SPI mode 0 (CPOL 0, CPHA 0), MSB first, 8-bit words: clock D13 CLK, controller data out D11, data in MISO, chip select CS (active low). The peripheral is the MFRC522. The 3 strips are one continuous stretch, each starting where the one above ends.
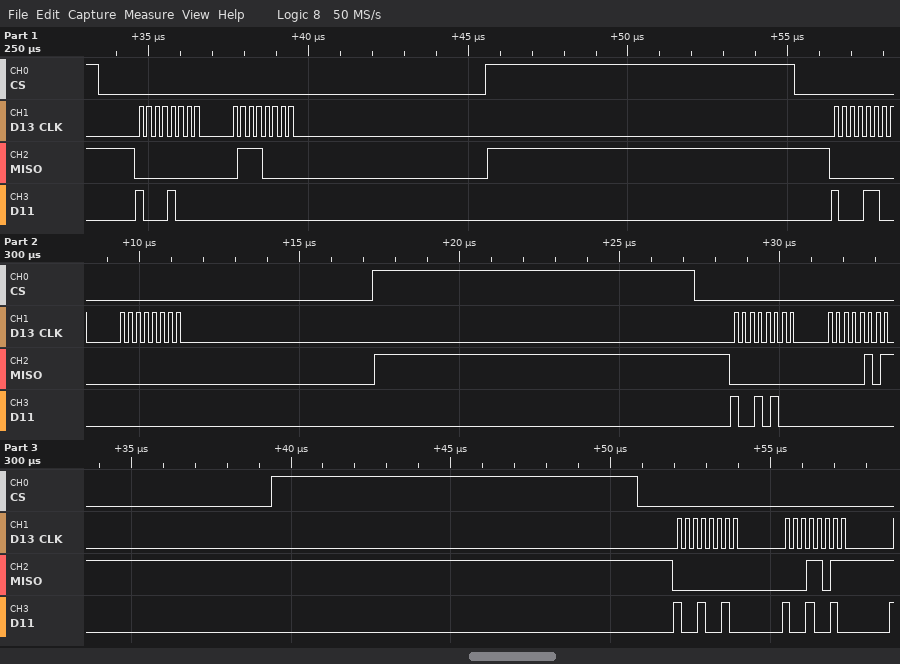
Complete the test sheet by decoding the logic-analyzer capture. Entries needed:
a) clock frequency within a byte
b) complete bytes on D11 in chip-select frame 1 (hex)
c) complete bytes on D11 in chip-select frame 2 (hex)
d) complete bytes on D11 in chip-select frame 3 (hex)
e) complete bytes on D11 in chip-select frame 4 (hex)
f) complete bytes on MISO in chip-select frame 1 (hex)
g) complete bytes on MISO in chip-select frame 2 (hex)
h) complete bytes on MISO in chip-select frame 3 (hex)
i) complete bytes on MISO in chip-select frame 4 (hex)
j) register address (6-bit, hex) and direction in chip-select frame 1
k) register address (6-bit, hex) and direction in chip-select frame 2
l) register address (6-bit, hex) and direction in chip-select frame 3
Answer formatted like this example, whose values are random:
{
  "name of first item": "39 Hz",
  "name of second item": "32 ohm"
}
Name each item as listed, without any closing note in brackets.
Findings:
{
  "clock frequency within a byte": "4 MHz",
  "complete bytes on D11 in chip-select frame 1": "88 00",
  "complete bytes on D11 in chip-select frame 2": "8C 00",
  "complete bytes on D11 in chip-select frame 3": "94 00",
  "complete bytes on D11 in chip-select frame 4": "92 92",
  "complete bytes on MISO in chip-select frame 1": "00 70",
  "complete bytes on MISO in chip-select frame 2": "00 00",
  "complete bytes on MISO in chip-select frame 3": "00 05",
  "complete bytes on MISO in chip-select frame 4": "00 1B",
  "register address (6-bit, hex) and direction in chip-select frame 1": "0x04 read",
  "register address (6-bit, hex) and direction in chip-select frame 2": "0x06 read",
  "register address (6-bit, hex) and direction in chip-select frame 3": "0x0A read"
}
